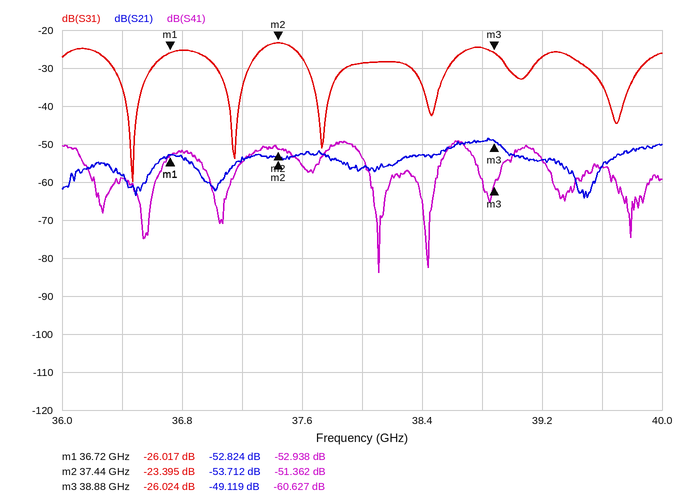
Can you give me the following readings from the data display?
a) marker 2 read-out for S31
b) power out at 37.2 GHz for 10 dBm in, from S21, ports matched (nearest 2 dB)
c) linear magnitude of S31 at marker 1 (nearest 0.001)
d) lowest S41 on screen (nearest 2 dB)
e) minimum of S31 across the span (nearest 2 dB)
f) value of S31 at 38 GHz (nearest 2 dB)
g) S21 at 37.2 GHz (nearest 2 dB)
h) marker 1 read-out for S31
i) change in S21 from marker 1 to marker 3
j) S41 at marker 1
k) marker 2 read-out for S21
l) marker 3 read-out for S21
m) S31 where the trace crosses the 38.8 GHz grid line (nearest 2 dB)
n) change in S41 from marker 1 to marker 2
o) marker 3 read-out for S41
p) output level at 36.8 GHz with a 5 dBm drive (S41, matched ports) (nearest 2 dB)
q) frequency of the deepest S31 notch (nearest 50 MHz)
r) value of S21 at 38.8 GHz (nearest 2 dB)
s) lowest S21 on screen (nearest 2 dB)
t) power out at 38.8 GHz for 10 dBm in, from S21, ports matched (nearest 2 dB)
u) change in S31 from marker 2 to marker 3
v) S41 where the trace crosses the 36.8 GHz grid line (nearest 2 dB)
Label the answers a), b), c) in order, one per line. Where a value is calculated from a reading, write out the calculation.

a) -23.395 dB
b) 10 dBm + (-54 dB) = -44 dBm
c) 10^(-26.017/20) ≈ 0.050
d) -84 dB
e) -60 dB
f) -28 dB
g) -54 dB
h) -26.017 dB
i) -49.119 − (-52.824) = 3.705 dB
j) -52.938 dB
k) -53.712 dB
l) -49.119 dB
m) -24 dB
n) -51.362 − (-52.938) = 1.576 dB
o) -60.627 dB
p) 5 dBm + (-52 dB) = -46 dBm
q) 36.45 GHz
r) -50 dB
s) -64 dB
t) 10 dBm + (-50 dB) = -40 dBm
u) -26.024 − (-23.395) = -2.629 dB
v) -52 dB
